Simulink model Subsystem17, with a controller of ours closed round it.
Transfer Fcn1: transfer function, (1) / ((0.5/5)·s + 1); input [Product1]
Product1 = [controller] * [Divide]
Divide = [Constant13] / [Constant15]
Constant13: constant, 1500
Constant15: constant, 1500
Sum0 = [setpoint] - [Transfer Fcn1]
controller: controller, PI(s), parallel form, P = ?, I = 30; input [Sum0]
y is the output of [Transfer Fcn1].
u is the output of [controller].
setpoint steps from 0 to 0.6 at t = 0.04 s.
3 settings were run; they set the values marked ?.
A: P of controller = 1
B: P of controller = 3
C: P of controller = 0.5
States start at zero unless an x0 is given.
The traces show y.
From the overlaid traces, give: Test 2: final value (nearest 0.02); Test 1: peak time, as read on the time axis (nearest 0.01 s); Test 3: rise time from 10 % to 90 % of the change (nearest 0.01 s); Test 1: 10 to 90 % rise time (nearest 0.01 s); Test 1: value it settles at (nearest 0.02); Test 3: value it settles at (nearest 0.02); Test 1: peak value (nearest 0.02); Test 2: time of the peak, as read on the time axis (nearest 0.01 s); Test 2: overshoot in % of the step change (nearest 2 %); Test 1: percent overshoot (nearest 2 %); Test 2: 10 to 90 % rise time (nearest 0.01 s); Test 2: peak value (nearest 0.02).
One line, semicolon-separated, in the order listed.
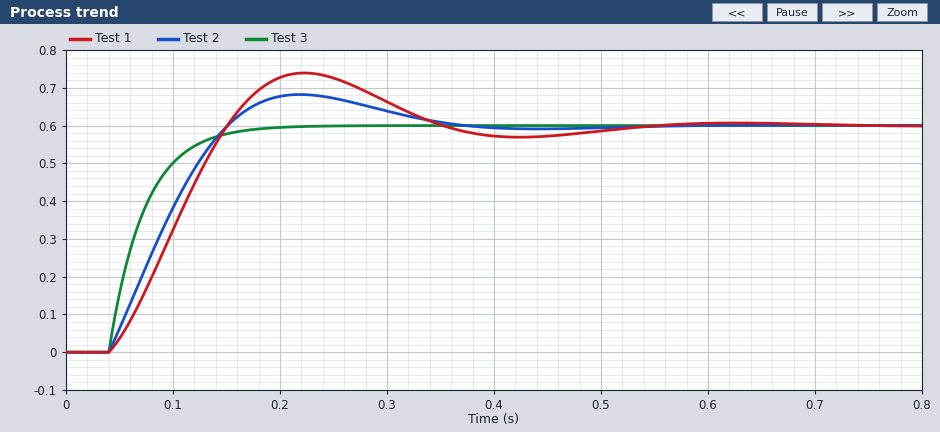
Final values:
0.60; 0.22 s; 0.07 s; 0.08 s; 0.60; 0.60; 0.74; 0.22 s; 14 %; 24 %; 0.08 s; 0.68
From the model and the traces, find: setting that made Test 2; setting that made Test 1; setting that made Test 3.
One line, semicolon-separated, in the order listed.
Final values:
A; C; B
